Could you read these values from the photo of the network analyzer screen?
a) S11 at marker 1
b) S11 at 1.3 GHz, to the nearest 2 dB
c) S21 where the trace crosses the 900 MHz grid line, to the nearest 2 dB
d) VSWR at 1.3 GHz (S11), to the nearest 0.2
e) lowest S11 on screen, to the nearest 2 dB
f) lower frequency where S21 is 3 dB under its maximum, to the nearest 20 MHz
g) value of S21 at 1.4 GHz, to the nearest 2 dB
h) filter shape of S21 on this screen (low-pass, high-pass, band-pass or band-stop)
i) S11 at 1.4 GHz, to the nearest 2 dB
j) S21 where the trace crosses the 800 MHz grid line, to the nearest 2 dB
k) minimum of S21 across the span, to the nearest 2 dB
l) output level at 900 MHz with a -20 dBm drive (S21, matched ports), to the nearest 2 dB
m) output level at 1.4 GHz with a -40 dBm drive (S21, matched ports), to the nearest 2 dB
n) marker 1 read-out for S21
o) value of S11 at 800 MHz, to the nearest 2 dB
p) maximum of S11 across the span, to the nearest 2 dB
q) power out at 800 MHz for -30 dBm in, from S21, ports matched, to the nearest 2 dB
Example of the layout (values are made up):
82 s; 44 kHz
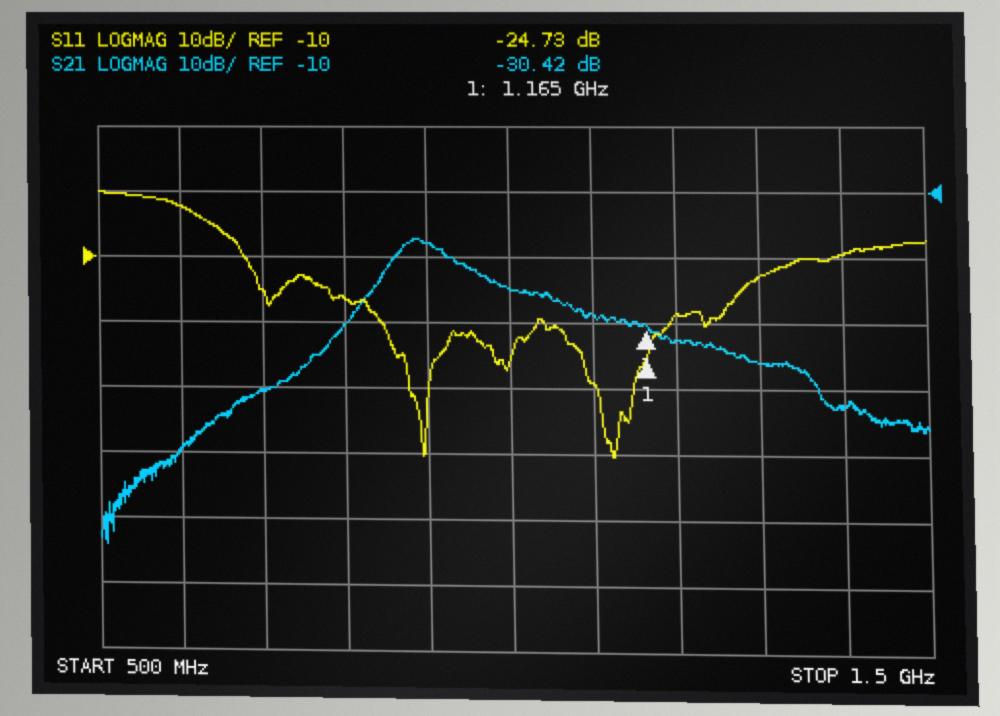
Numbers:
-24.73 dB; -12 dB; -18 dB; 1.6; -40 dB; 860 MHz; -42 dB; band-pass; -10 dB; -30 dB; -64 dB; -38 dBm; -82 dBm; -30.42 dB; -16 dB; 0 dB; -60 dBm
